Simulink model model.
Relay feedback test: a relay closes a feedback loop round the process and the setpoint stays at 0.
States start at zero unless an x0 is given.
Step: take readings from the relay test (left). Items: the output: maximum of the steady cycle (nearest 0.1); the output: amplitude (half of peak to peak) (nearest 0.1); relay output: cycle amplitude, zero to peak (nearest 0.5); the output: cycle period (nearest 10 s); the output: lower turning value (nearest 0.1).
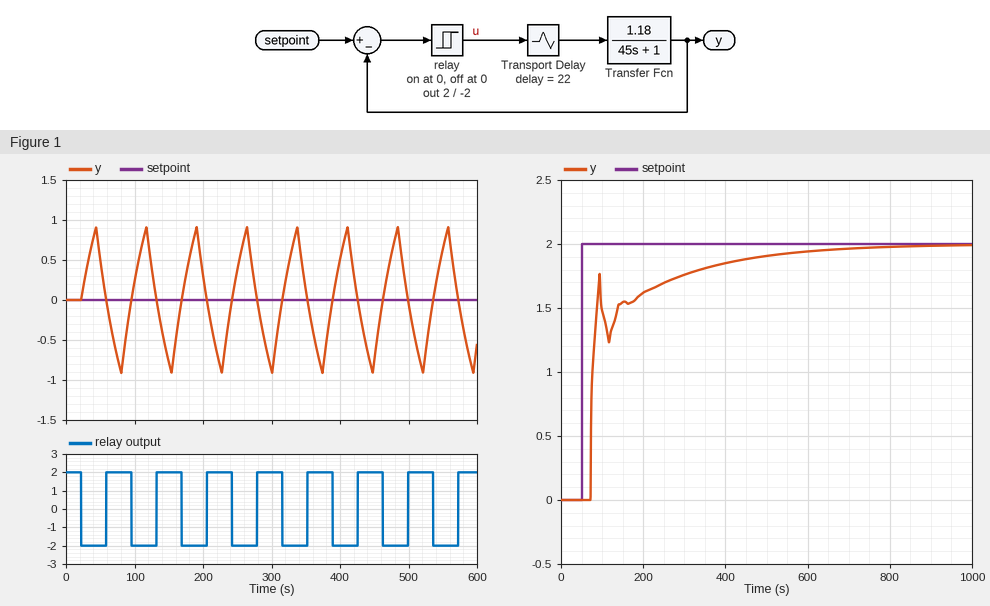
0.9
0.9
2.0
70 s
-0.9
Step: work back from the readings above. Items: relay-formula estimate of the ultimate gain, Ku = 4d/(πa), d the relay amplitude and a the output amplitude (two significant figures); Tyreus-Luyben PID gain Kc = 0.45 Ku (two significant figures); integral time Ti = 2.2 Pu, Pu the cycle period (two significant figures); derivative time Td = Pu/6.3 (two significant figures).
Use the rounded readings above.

2.8
1.3
150 s
11 s
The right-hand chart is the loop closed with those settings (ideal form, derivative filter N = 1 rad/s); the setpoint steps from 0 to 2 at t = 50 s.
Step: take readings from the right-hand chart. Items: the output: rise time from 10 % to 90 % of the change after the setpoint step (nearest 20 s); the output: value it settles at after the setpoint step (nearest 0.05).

260 s
2.00
